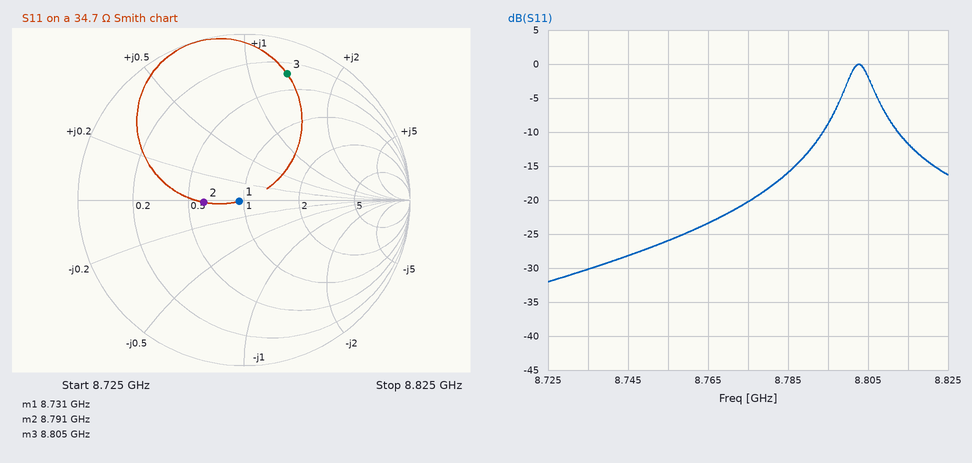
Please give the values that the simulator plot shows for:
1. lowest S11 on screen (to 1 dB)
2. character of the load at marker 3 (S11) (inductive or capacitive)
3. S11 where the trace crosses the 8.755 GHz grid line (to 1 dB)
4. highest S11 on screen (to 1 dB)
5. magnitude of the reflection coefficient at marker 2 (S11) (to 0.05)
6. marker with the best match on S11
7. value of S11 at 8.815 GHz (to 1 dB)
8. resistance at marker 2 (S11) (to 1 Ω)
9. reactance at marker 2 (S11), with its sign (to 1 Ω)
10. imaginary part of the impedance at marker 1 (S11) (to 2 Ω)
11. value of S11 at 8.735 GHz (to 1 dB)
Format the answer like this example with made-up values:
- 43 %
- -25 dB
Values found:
- -32 dB
- inductive
- -26 dB
- 0 dB
- 0.25
- marker 1
- -12 dB
- 21 Ω
- -1 Ω
- 0 Ω
- -30 dB
